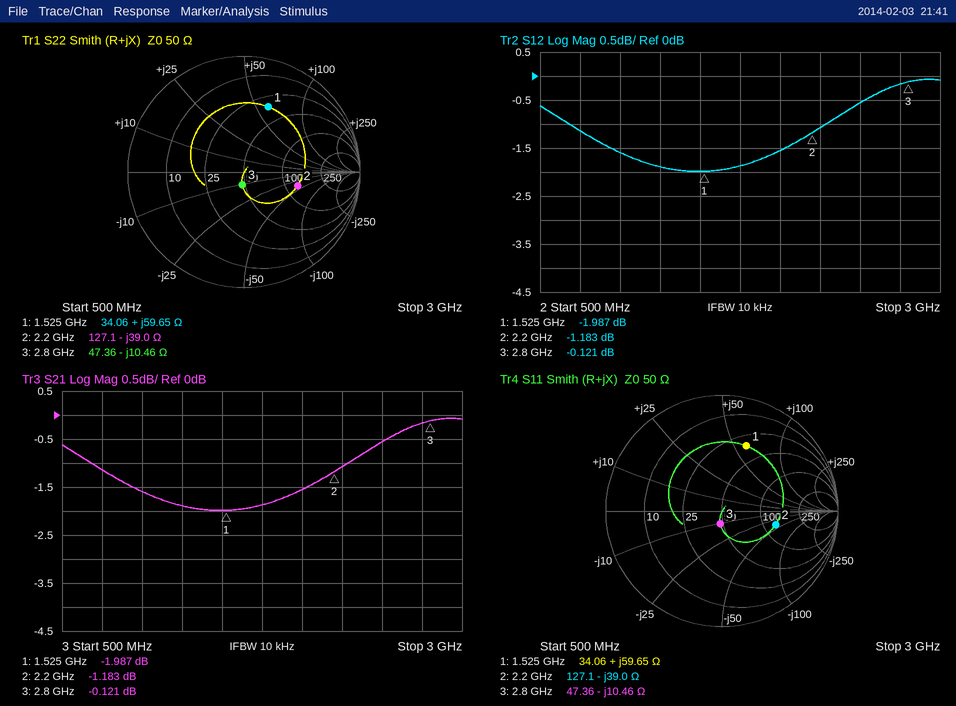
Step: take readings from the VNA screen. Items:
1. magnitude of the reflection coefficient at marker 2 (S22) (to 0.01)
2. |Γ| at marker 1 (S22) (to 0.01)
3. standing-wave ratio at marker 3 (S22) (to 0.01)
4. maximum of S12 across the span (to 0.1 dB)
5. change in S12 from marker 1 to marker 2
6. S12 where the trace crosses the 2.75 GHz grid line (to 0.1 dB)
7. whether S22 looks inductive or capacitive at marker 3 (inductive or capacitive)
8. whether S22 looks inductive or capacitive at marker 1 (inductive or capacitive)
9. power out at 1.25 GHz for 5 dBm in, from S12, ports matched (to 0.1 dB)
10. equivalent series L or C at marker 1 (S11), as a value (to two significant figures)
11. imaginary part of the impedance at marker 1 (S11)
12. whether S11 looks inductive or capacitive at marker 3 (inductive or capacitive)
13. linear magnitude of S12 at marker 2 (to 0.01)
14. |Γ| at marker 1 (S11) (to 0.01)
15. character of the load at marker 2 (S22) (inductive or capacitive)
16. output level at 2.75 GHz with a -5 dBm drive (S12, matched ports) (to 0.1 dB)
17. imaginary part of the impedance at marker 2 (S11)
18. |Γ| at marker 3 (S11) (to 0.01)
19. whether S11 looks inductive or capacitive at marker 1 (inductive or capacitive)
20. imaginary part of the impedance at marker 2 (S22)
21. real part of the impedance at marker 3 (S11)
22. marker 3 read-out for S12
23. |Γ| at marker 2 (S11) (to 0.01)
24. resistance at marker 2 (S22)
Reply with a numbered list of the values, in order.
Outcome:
1. 0.48
2. 0.60
3. 1.25
4. -0.1 dB
5. 0.804 dB
6. -0.2 dB
7. capacitive
8. inductive
9. 3.1 dBm
10. 6.2 nH
11. +59.65 Ω
12. capacitive
13. 0.87
14. 0.60
15. capacitive
16. -5.2 dBm
17. -39.0 Ω
18. 0.11
19. inductive
20. -39.0 Ω
21. 47.36 Ω
22. -0.121 dB
23. 0.48
24. 127.1 Ω
